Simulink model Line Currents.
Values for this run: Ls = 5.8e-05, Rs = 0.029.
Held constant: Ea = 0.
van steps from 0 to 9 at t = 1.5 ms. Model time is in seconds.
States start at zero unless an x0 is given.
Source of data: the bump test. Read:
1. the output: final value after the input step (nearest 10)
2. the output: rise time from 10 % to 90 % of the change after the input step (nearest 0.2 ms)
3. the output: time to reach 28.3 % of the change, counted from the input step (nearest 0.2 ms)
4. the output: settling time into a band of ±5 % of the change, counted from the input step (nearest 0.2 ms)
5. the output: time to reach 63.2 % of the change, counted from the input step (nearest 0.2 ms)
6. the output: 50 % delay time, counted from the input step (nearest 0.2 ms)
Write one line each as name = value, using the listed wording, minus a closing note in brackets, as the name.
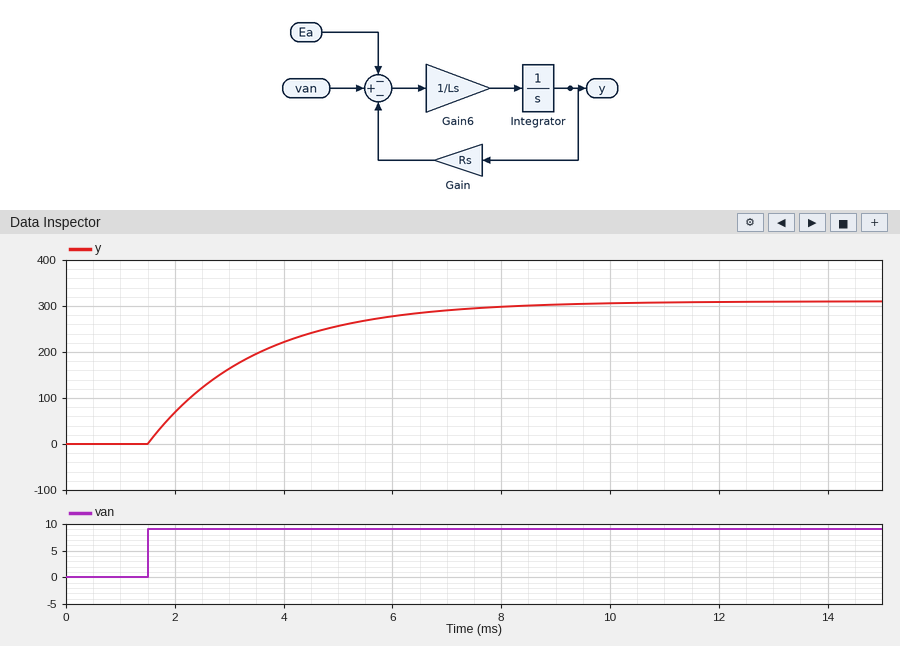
the output: final value after the input step = 310
the output: rise time from 10 % to 90 % of the change after the input step = 4.4 ms
the output: time to reach 28.3 % of the change, counted from the input step = 0.6 ms
the output: settling time into a band of ±5 % of the change, counted from the input step = 6.0 ms
the output: time to reach 63.2 % of the change, counted from the input step = 2.0 ms
the output: 50 % delay time, counted from the input step = 1.4 ms
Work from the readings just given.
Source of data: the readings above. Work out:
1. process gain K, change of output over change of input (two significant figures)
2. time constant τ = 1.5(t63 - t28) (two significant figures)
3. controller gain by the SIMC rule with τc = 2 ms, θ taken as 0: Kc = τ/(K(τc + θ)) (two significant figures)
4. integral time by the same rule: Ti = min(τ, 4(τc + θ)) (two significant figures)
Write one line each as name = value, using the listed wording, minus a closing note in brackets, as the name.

process gain K, change of output over change of input = 34
time constant τ = 1.5(t63 - t28) = 2.1 ms
controller gain by the SIMC rule with τc = 2 ms, θ taken as 0: Kc = τ/(K(τc + θ)) = 0.031
integral time by the same rule: Ti = min(τ, 4(τc + θ)) = 2.1 ms
